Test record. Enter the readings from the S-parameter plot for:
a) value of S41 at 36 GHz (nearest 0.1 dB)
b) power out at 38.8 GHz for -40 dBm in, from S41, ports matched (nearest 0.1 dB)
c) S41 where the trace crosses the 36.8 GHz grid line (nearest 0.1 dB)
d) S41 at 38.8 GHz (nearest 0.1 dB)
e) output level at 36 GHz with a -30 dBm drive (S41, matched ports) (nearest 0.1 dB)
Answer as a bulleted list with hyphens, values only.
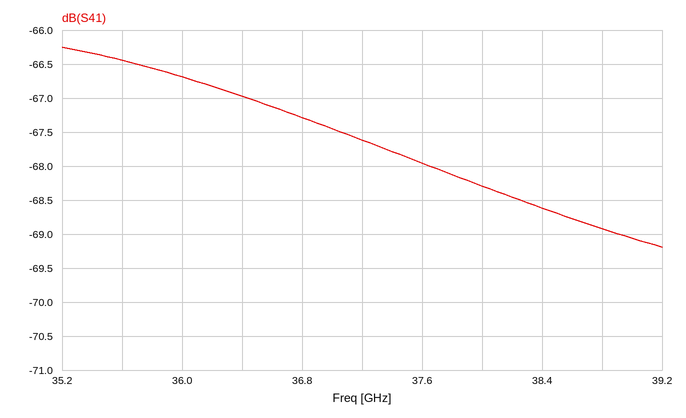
- -66.7 dB
- -108.9 dBm
- -67.3 dB
- -68.9 dB
- -96.7 dBm
